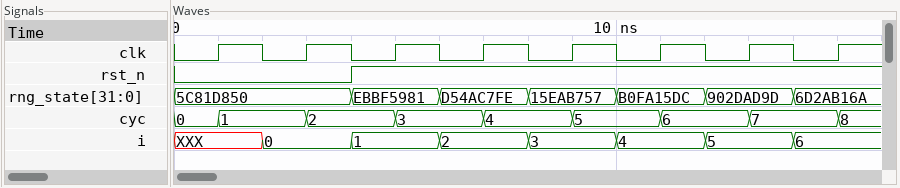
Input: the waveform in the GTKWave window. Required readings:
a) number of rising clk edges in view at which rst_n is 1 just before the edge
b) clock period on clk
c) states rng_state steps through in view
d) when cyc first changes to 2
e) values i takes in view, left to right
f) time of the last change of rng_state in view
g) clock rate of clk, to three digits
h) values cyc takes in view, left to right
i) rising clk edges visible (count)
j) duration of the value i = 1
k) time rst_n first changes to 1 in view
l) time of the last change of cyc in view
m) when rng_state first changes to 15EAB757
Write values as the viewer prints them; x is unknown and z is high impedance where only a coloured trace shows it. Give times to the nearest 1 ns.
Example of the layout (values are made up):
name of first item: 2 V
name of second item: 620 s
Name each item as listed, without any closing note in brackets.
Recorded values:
number of rising clk edges in view at which rst_n is 1 just before the edge: 6
clock period on clk: 2 ns
states rng_state steps through in view: 5C81D850, EBBF5981, D54AC7FE, 15EAB757, B0FA15DC, 902DAD9D, 6D2AB16A
when cyc first changes to 2: 3 ns
values i takes in view, left to right: XXX, 0, 1, 2, 3, 4, 5, 6
time of the last change of rng_state in view: 14 ns
clock rate of clk, to three digits: 500 MHz
values cyc takes in view, left to right: 0, 1, 2, 3, 4, 5, 6, 7, 8
rising clk edges visible: 8
duration of the value i = 1: 2 ns
time rst_n first changes to 1 in view: 4 ns
time of the last change of cyc in view: 15 ns
when rng_state first changes to 15EAB757: 8 ns
